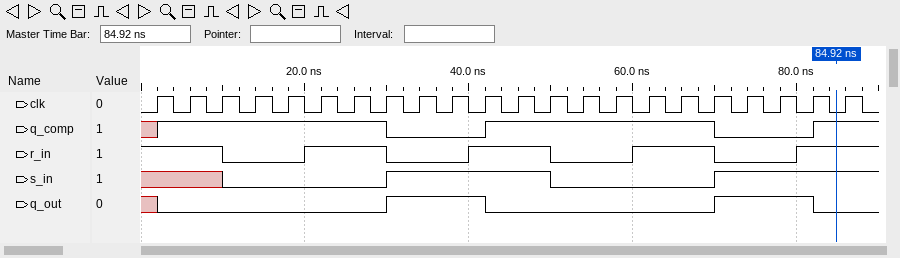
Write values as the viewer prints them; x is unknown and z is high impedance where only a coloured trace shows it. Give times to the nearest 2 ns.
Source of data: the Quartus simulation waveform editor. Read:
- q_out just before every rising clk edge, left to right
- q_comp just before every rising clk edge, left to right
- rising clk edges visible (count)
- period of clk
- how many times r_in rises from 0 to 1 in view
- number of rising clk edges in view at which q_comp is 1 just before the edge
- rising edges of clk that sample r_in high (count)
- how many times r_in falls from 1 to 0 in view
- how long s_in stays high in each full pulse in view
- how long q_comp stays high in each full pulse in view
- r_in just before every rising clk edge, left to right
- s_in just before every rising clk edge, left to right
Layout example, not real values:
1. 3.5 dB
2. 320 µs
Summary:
1. x 0 0 0 0 0 0 0 1 1 1 0 0 0 0 0 0 0 1 1 1 0
2. x 1 1 1 1 1 1 1 0 0 0 1 1 1 1 1 1 1 0 0 0 1
3. 22
4. 4 ns
5. 4
6. 15
7. 14
8. 4
9. 20 ns
10. 28 ns
11. 1 1 1 0 0 1 1 1 0 0 1 1 1 0 0 1 1 1 0 0 1 1
12. x x x 0 0 0 0 0 1 1 1 1 1 0 0 0 0 0 1 1 1 1
